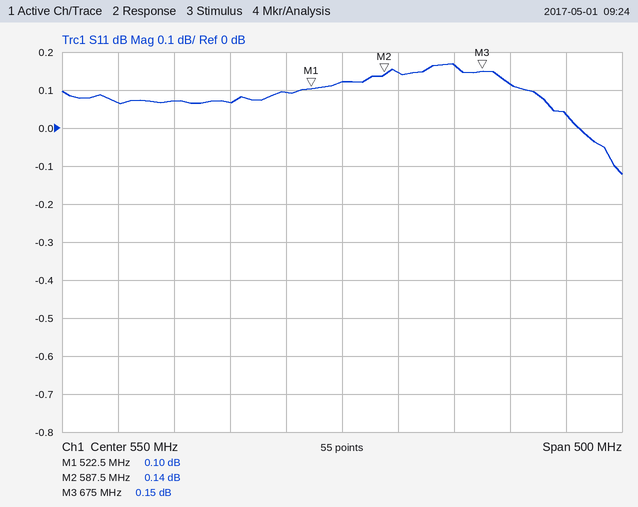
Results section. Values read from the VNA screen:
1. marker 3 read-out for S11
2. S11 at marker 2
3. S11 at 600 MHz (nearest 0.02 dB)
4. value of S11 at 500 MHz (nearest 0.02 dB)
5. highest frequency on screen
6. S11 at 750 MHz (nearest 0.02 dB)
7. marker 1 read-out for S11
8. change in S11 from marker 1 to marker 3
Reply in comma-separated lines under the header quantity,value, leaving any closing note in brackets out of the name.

quantity,value
marker 3 read-out for S11,0.15 dB
S11 at marker 2,0.14 dB
S11 at 600 MHz,0.14 dB
value of S11 at 500 MHz,0.10 dB
highest frequency on screen,800 MHz
S11 at 750 MHz,0.04 dB
marker 1 read-out for S11,0.10 dB
change in S11 from marker 1 to marker 3,0.05 dB
